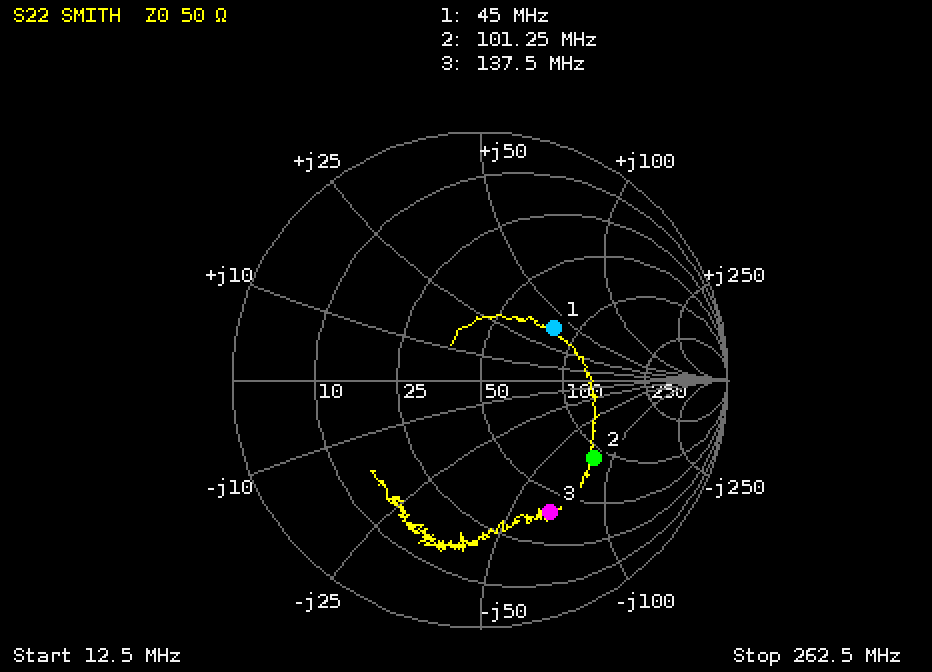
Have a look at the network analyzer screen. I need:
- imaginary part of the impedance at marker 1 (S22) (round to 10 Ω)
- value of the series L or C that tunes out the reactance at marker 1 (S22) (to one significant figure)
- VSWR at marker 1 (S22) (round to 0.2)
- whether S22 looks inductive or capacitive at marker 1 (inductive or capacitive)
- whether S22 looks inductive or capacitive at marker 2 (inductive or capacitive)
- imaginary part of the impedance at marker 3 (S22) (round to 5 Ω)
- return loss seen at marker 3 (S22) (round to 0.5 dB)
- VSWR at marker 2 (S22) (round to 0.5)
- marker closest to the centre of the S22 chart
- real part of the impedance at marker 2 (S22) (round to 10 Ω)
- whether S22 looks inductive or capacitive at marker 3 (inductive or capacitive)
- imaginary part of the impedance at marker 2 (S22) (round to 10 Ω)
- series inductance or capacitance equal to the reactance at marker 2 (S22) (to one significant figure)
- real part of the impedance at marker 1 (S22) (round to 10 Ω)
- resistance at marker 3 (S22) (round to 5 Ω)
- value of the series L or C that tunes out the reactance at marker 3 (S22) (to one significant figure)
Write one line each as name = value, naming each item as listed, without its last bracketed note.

imaginary part of the impedance at marker 1 (S22) = +40 Ω
value of the series L or C that tunes out the reactance at marker 1 (S22) = 90 pF
VSWR at marker 1 (S22) = 2.2
whether S22 looks inductive or capacitive at marker 1 = inductive
whether S22 looks inductive or capacitive at marker 2 = capacitive
imaginary part of the impedance at marker 3 (S22) = -65 Ω
return loss seen at marker 3 (S22) = 4.5 dB
VSWR at marker 2 (S22) = 3.5
marker closest to the centre of the S22 chart = marker 1
real part of the impedance at marker 2 (S22) = 90 Ω
whether S22 looks inductive or capacitive at marker 3 = capacitive
imaginary part of the impedance at marker 2 (S22) = -80 Ω
series inductance or capacitance equal to the reactance at marker 2 (S22) = 20 pF
real part of the impedance at marker 1 (S22) = 80 Ω
resistance at marker 3 (S22) = 40 Ω
value of the series L or C that tunes out the reactance at marker 3 (S22) = 80 nH
